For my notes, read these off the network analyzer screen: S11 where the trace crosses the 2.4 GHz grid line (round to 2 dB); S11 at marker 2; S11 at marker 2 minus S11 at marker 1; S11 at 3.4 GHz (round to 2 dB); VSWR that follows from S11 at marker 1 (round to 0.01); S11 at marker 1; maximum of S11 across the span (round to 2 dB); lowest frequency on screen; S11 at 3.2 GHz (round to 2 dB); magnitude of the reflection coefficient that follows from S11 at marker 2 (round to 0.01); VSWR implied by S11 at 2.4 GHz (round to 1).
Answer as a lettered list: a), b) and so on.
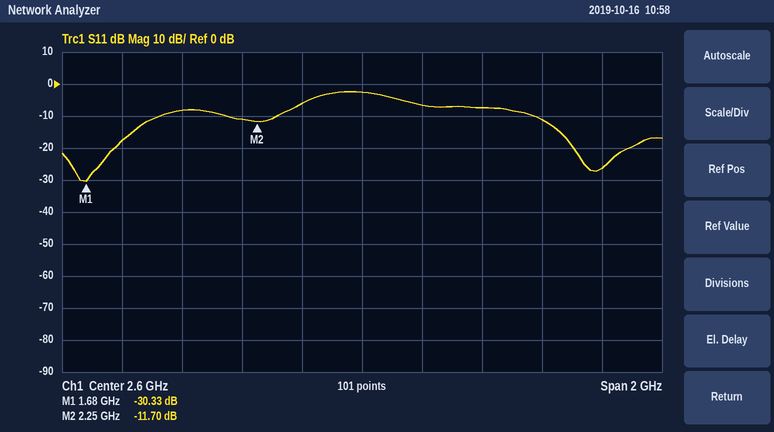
a) -6 dB
b) -11.70 dB
c) 18.63 dB
d) -26 dB
e) 1.06
f) -30.33 dB
g) -2 dB
h) 1.6 GHz
i) -12 dB
j) 0.26
k) 3
